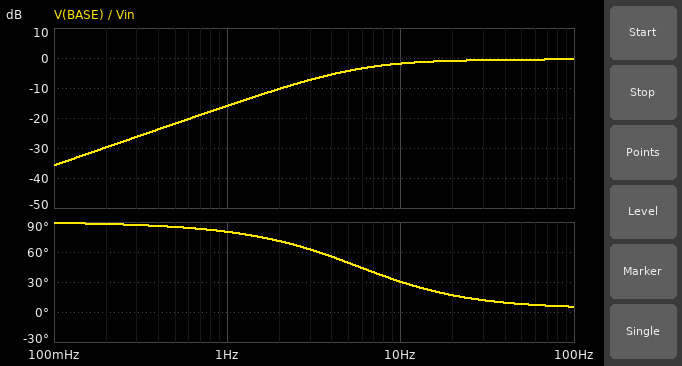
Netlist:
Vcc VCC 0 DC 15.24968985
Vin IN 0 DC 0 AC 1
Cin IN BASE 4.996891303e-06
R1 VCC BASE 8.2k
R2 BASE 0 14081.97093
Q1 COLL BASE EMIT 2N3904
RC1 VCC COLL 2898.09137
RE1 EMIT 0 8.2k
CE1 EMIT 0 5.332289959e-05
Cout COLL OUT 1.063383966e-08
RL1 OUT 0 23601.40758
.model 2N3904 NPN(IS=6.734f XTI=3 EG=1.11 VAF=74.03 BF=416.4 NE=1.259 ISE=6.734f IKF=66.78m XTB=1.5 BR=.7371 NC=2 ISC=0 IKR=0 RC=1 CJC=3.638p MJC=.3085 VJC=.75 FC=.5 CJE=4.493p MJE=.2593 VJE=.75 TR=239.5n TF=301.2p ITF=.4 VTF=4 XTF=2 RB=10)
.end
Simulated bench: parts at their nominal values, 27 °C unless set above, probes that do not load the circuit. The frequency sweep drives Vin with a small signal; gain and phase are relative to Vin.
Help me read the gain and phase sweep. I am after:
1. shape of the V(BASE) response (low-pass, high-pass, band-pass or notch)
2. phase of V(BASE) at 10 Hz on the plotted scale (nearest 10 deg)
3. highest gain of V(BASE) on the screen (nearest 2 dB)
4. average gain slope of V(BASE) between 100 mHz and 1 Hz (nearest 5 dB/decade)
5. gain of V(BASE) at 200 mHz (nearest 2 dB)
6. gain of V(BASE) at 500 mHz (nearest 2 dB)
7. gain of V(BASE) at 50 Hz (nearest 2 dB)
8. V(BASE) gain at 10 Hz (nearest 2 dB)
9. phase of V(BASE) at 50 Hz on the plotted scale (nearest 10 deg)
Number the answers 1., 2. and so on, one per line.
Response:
1. high-pass
2. 30 deg
3. 0 dB
4. 20 dB/decade
5. -30 dB
6. -22 dB
7. 0 dB
8. -2 dB
9. 10 deg
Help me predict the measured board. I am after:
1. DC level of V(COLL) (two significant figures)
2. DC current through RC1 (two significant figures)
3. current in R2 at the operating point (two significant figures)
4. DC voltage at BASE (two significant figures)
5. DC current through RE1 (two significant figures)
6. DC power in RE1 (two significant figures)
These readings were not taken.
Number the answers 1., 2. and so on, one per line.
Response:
1. 12 V
2. 1.1 mA
3. 680 µA
4. 9.6 V
5. 1.1 mA
6. 9.7 mW
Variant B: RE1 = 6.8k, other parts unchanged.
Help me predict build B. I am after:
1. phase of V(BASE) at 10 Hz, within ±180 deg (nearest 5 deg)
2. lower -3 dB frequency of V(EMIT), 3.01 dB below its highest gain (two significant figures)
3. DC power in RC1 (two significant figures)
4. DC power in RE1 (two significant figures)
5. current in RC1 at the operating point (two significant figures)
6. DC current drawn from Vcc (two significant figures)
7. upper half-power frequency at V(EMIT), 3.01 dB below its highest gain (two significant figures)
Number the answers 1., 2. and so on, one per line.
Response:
1. 30 deg
2. 5.4 Hz
3. 4.9 mW
4. 12 mW
5. 1.3 mA
6. 2.0 mA
7. 160 Hz
